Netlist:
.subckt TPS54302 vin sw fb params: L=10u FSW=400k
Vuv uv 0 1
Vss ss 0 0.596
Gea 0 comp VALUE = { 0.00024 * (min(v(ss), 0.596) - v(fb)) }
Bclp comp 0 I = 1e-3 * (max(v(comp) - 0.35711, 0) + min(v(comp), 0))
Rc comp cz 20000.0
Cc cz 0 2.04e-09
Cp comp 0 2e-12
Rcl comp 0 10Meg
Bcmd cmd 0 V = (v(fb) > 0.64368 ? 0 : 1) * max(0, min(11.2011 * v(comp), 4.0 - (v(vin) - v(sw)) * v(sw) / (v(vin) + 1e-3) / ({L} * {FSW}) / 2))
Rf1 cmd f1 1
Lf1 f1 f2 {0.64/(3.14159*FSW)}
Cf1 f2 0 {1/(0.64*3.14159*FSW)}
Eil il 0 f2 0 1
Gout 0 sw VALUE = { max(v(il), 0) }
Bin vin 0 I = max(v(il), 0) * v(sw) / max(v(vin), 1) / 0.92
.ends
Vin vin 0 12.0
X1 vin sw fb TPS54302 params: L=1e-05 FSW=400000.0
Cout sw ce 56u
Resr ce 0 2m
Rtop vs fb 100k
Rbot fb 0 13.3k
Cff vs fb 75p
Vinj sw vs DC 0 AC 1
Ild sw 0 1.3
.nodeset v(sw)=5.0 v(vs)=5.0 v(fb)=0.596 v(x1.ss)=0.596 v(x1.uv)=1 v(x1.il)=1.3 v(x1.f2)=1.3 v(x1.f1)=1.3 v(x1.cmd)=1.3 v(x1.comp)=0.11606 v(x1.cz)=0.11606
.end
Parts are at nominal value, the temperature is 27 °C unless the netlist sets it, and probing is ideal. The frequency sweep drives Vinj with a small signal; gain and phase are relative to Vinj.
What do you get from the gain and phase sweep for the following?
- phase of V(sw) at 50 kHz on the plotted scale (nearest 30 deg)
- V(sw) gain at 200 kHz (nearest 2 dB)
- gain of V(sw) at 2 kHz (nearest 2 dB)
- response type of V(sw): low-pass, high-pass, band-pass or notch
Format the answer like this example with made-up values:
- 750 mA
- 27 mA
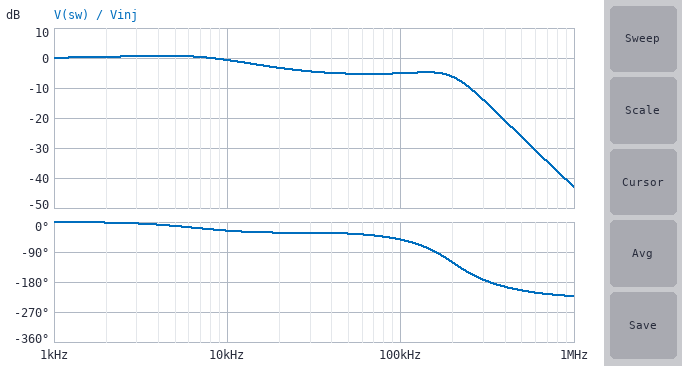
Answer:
- -30 deg
- -6 dB
- 0 dB
- low-pass
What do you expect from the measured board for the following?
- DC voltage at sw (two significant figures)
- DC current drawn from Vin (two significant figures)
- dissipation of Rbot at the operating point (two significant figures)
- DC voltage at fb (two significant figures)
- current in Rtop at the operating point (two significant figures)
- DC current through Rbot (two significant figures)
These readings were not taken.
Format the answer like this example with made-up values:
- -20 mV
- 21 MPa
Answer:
- 5.1 V
- 600 mA
- 27 µW
- 600 mV
- 45 µA
- 45 µA
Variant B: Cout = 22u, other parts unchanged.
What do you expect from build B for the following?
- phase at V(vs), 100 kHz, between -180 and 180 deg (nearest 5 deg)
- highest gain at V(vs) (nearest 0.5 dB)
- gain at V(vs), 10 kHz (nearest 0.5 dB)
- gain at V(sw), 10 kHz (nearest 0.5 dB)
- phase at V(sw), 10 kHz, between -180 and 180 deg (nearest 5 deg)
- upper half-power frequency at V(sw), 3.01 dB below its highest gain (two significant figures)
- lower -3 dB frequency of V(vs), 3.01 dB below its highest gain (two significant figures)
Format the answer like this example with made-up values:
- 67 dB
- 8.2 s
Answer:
- -120 deg
- 7.5 dB
- -14.5 dB
- 0 dB
- -10 deg
- 260 kHz
- 200 kHz
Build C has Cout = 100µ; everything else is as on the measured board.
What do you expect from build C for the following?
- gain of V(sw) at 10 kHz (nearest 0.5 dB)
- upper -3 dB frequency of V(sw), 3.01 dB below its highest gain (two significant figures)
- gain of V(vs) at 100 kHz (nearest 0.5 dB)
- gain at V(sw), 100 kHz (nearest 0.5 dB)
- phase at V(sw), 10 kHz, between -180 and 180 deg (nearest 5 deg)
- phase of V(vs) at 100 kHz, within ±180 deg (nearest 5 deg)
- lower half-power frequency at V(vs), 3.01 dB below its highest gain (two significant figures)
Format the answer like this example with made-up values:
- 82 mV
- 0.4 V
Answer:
- -2.0 dB
- 9.4 kHz
- -1.0 dB
- -9.0 dB
- -40 deg
- -160 deg
- 72 kHz
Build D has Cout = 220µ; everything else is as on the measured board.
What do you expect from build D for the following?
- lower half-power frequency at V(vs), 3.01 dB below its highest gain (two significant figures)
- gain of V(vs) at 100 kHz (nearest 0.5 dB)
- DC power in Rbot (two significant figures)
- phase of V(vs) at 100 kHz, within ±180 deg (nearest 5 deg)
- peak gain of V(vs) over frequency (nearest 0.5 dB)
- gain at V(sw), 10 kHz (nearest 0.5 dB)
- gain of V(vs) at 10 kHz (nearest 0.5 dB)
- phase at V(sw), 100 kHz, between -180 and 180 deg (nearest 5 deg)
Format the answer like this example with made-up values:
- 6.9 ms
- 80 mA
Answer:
- 3.9 kHz
- -0.5 dB
- 27 µW
- -170 deg
- 0.5 dB
- -6.5 dB
- -1.0 dB
- -65 deg
